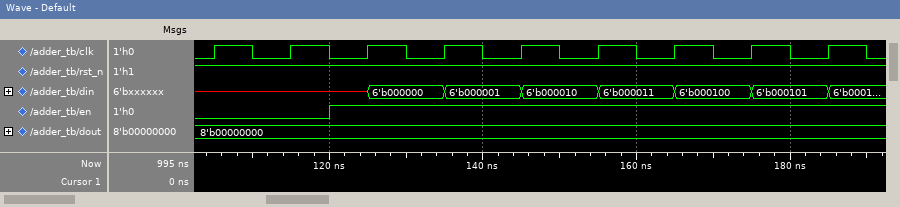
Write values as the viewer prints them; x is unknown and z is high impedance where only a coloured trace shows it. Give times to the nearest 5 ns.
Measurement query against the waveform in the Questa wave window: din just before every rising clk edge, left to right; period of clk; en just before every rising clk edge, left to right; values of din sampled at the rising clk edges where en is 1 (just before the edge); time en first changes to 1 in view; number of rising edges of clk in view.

x, x, x, 6'b000000, 6'b000001, 6'b000010, 6'b000011, 6'b000100, 6'b000101
10 ns
0 0 1 1 1 1 1 1 1
x, 6'b000000, 6'b000001, 6'b000010, 6'b000011, 6'b000100, 6'b000101
120 ns
9
